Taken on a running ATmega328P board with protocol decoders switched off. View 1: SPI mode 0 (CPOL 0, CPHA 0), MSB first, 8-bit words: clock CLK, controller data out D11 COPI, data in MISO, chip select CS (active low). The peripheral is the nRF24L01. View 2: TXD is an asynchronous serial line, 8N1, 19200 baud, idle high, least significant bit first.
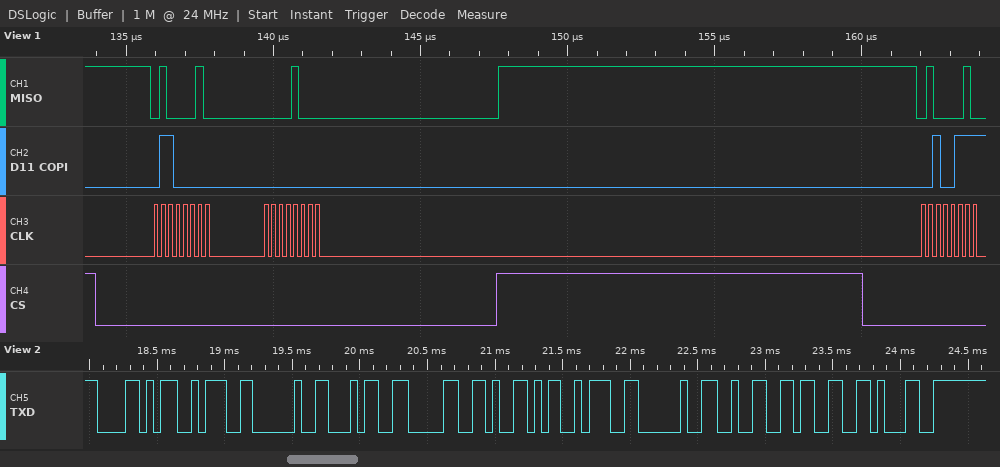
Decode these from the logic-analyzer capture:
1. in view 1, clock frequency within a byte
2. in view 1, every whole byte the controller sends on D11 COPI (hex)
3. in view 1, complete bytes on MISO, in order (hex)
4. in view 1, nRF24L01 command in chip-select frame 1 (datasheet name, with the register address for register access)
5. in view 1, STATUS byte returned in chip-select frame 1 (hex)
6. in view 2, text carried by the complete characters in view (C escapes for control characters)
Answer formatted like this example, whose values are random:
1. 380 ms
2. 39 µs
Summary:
1. 4 MHz
2. 0x60 0x00 0x27
3. 0x42 0x08 0x42
4. R_RX_PL_WID
5. 0x42
6. "X: 40Y: 231"
